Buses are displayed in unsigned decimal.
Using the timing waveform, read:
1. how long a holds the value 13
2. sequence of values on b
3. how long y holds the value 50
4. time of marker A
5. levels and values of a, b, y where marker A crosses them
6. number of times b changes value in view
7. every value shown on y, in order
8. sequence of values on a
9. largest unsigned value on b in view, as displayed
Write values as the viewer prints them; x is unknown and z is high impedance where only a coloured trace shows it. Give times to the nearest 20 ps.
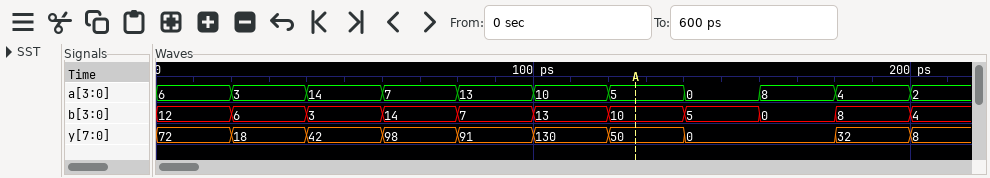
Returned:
20 ps
12, 6, 3, 14, 7, 13, 10, 5, 0, 8, 4
20 ps
120 ps
a=5, b=10, y=50
10
72, 18, 42, 98, 91, 130, 50, 0, 32, 8
6, 3, 14, 7, 13, 10, 5, 0, 8, 4, 2
14
